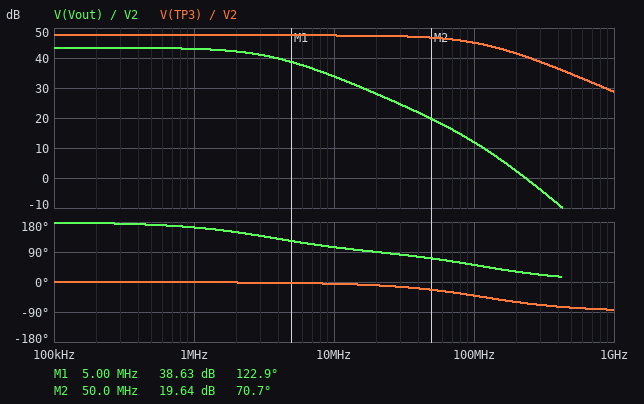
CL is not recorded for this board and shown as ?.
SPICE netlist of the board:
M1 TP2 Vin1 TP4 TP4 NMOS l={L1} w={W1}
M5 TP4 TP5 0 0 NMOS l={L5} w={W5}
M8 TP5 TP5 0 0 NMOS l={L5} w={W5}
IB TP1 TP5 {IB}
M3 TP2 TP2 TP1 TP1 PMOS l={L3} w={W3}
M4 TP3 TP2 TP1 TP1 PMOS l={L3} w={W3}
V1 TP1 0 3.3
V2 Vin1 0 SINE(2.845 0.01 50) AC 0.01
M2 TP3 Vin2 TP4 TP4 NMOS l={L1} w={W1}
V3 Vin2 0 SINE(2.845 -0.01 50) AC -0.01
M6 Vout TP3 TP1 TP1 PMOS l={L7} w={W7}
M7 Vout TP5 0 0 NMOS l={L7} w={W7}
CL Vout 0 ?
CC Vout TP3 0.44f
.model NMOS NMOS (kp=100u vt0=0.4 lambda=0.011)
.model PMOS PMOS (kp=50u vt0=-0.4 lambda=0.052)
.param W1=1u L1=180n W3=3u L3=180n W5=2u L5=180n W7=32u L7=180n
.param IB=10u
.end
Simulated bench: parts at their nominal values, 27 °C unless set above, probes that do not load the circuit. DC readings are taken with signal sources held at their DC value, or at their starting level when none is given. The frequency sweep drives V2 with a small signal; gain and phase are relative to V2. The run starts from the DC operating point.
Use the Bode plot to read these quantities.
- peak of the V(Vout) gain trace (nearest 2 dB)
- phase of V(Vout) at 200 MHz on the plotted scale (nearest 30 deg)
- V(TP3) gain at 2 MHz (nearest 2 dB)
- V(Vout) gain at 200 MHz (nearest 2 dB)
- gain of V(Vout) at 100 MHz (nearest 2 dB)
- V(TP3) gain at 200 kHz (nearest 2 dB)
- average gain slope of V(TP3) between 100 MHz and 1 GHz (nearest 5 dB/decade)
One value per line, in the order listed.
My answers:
44 dB
30 deg
48 dB
2 dB
12 dB
48 dB
-15 dB/decade
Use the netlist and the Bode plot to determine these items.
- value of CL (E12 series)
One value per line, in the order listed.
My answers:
82 pF
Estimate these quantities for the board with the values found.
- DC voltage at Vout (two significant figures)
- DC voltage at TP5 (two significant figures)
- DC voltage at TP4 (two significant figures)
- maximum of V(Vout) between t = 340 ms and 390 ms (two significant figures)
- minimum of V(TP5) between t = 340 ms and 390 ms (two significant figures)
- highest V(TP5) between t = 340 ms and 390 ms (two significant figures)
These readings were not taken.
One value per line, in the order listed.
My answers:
29 mV
530 mV
2.3 V
3.3 V
530 mV
530 mV
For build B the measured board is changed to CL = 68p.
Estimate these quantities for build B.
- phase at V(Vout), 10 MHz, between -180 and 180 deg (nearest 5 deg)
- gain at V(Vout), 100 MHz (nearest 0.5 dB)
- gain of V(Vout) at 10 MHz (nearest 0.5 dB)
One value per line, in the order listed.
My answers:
110 deg
13.5 dB
35.0 dB
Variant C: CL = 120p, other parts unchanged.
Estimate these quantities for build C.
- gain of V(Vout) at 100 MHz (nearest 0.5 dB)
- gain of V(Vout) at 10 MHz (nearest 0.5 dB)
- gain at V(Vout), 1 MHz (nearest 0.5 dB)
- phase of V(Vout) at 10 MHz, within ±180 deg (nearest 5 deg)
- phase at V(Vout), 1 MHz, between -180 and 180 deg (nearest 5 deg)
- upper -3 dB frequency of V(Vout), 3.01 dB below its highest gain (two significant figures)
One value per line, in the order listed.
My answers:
8.5 dB
31.0 dB
42.5 dB
100 deg
155 deg
2.4 MHz
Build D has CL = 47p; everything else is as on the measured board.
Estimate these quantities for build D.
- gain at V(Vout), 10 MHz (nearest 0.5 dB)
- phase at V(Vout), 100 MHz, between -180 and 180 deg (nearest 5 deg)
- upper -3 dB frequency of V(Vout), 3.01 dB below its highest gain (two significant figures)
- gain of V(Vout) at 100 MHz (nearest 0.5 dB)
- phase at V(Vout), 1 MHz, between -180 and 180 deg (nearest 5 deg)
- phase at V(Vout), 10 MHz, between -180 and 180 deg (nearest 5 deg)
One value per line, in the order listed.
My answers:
37.5 dB
55 deg
6.1 MHz
16.5 dB
170 deg
115 deg
